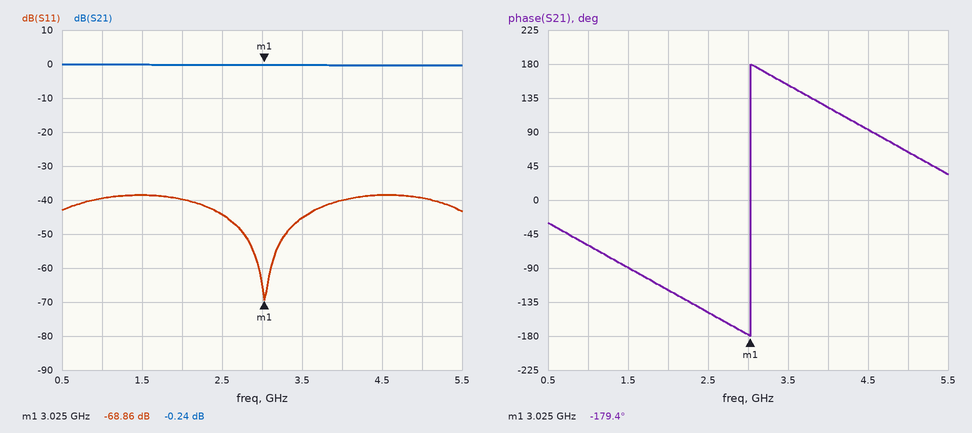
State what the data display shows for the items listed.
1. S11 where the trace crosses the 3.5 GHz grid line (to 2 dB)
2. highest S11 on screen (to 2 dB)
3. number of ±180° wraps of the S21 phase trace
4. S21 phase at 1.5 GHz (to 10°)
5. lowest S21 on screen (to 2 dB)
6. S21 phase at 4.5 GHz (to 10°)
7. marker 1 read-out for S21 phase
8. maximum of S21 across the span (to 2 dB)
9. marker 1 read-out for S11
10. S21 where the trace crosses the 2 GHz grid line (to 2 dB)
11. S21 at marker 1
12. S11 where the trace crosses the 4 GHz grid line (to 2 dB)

-46 dB
-38 dB
1
-90°
0 dB
90°
-179.4°
0 dB
-68.86 dB
0 dB
-0.24 dB
-40 dB
